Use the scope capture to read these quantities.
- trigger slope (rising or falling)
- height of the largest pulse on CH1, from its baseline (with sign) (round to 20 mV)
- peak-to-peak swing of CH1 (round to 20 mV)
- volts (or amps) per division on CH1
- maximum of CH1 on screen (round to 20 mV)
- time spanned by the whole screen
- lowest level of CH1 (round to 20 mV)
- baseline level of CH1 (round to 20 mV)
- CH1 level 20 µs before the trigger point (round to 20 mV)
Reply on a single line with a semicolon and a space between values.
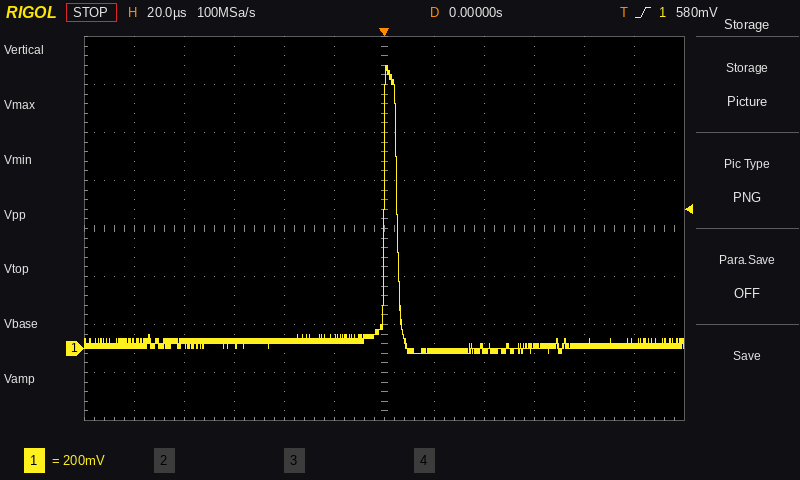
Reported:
rising; +1.16 V; 1.20 V; 200 mV; 1.18 V; 240 µs; -20 mV; 20 mV; 40 mV
